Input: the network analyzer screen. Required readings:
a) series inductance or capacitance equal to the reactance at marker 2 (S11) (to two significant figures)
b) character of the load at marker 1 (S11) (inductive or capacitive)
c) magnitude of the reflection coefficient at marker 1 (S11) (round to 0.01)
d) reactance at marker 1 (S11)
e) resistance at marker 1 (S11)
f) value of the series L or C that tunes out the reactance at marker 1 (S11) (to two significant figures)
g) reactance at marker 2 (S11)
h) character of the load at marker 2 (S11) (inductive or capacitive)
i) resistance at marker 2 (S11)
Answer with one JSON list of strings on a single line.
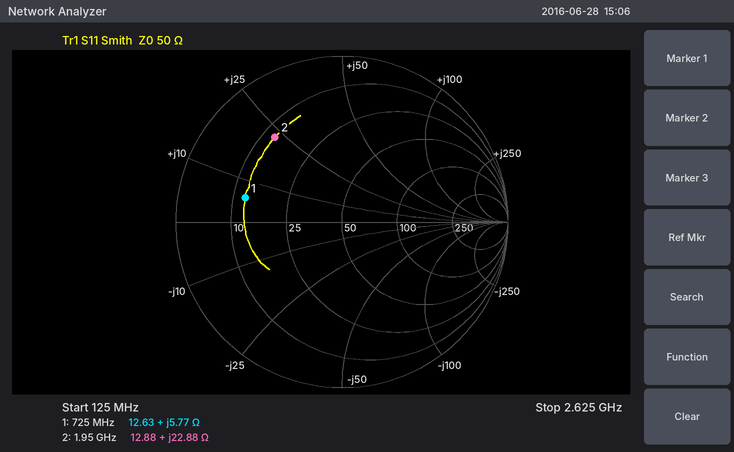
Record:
["1.9 nH", "inductive", "0.60", "+5.77 Ω", "12.63 Ω", "38 pF", "+22.88 Ω", "inductive", "12.88 Ω"]
